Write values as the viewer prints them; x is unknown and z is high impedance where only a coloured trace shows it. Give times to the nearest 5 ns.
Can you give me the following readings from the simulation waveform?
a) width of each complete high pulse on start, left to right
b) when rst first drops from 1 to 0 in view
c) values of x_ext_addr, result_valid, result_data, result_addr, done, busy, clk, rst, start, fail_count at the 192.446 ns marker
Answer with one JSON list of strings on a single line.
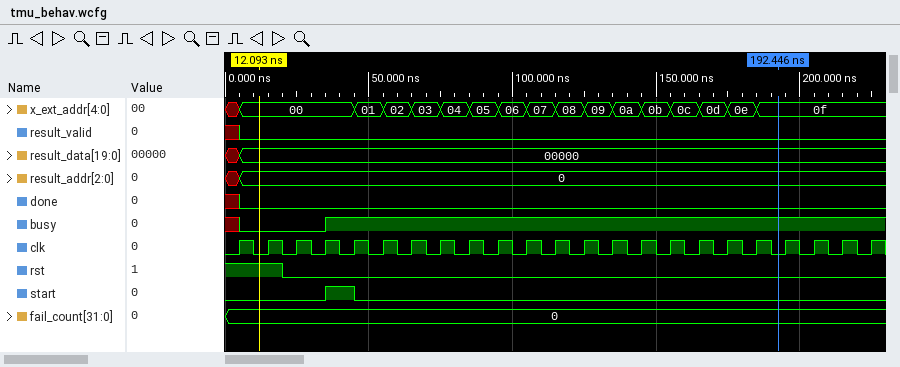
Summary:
["10 ns", "20 ns", "x_ext_addr=0f, result_valid=0, result_data=00000, result_addr=0, done=0, busy=1, clk=0, rst=0, start=0, fail_count=0"]
